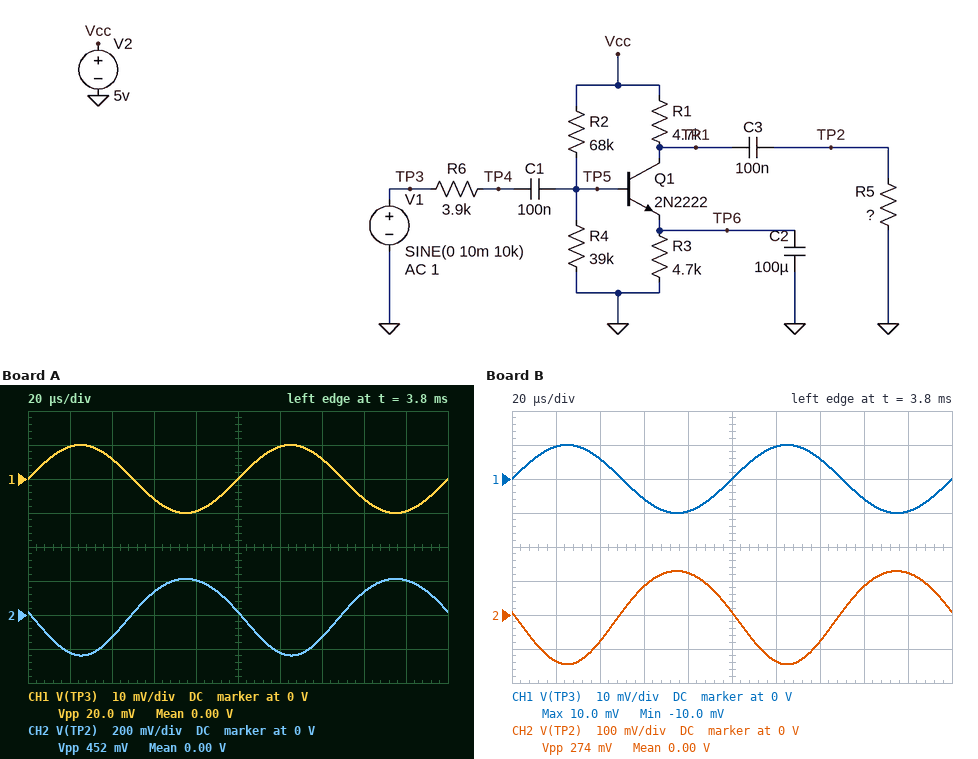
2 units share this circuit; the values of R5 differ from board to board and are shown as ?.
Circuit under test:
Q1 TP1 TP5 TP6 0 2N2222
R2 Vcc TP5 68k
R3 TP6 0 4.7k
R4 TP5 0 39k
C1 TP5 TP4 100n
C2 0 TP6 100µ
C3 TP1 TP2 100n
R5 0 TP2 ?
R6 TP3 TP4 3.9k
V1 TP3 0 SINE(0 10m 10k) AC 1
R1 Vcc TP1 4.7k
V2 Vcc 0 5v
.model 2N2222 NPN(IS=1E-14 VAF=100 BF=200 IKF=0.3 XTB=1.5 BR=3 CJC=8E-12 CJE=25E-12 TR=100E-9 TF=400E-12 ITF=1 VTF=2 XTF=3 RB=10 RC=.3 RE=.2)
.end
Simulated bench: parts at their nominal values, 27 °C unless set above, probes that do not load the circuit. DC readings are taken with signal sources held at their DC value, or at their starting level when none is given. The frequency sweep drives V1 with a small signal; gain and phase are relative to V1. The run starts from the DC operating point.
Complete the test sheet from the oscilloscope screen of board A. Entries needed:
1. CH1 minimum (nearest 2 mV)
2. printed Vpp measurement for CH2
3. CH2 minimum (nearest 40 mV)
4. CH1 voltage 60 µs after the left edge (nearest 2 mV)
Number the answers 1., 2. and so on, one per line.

1. -10 mV
2. 452 mV
3. -240 mV
4. -6 mV
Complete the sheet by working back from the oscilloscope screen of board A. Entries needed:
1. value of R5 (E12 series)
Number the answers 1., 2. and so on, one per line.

1. 10 kΩ
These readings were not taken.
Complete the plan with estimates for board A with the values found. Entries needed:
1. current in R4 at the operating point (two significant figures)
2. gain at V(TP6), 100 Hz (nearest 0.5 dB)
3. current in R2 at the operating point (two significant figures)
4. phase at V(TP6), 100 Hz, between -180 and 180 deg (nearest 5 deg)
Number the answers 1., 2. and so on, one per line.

1. 46 µA
2. -22.5 dB
3. 47 µA
4. -40 deg
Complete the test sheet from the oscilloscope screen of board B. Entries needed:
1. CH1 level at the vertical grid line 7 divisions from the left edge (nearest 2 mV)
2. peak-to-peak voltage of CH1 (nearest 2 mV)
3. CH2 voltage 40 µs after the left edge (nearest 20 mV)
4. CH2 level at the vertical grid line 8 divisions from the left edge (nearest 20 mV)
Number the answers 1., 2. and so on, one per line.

1. 6 mV
2. 20 mV
3. -80 mV
4. 80 mV
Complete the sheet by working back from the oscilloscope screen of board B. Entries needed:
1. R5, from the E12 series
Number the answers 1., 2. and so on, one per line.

1. 3.3 kΩ
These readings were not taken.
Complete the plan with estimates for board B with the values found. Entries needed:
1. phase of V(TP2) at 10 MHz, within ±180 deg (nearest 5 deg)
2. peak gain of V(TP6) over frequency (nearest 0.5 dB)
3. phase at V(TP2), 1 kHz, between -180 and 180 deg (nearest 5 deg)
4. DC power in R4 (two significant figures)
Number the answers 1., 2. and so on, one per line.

1. 80 deg
2. -20.5 dB
3. -160 deg
4. 82 µW
